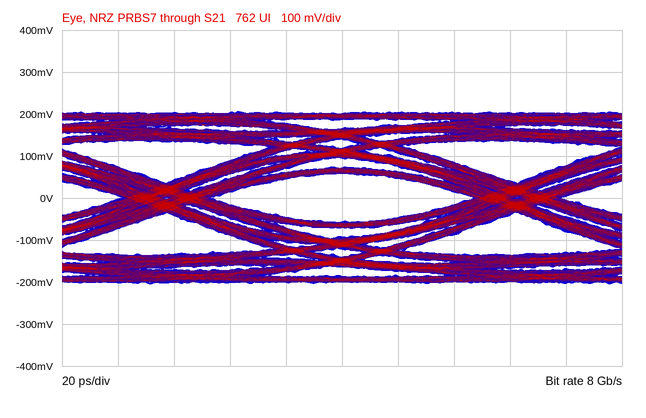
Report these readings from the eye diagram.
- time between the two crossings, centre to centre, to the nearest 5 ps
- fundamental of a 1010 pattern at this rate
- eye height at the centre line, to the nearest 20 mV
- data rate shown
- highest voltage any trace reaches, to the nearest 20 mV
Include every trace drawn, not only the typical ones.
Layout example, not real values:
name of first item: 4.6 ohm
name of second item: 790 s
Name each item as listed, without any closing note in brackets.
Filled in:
time between the two crossings, centre to centre, to the nearest 5 ps: 125 ps
fundamental of a 1010 pattern at this rate: 4 GHz
eye height at the centre line, to the nearest 20 mV: 120 mV
data rate shown: 8 Gb/s
highest voltage any trace reaches, to the nearest 20 mV: 200 mV
